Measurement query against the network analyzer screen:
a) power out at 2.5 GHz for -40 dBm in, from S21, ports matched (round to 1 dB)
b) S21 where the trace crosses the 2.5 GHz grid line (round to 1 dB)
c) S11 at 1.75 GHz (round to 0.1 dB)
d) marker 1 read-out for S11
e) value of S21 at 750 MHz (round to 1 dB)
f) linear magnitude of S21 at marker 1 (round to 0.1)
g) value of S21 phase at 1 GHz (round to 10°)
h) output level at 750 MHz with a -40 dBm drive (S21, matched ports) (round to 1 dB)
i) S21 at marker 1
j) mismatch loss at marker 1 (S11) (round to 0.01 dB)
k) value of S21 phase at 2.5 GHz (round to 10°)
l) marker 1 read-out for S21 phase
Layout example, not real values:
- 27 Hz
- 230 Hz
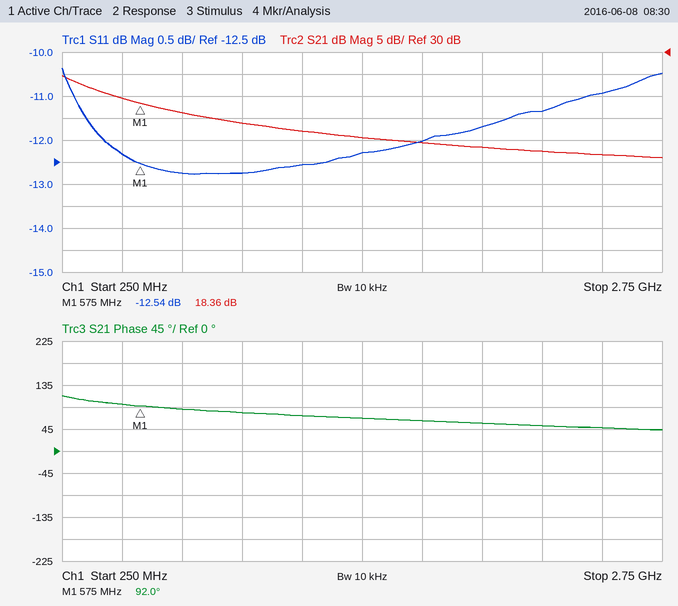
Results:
- -33 dBm
- 7 dB
- -12.0 dB
- -12.54 dB
- 16 dB
- 8.3
- 80°
- -24 dBm
- 18.36 dB
- 0.25 dB
- 50°
- 92.0°
